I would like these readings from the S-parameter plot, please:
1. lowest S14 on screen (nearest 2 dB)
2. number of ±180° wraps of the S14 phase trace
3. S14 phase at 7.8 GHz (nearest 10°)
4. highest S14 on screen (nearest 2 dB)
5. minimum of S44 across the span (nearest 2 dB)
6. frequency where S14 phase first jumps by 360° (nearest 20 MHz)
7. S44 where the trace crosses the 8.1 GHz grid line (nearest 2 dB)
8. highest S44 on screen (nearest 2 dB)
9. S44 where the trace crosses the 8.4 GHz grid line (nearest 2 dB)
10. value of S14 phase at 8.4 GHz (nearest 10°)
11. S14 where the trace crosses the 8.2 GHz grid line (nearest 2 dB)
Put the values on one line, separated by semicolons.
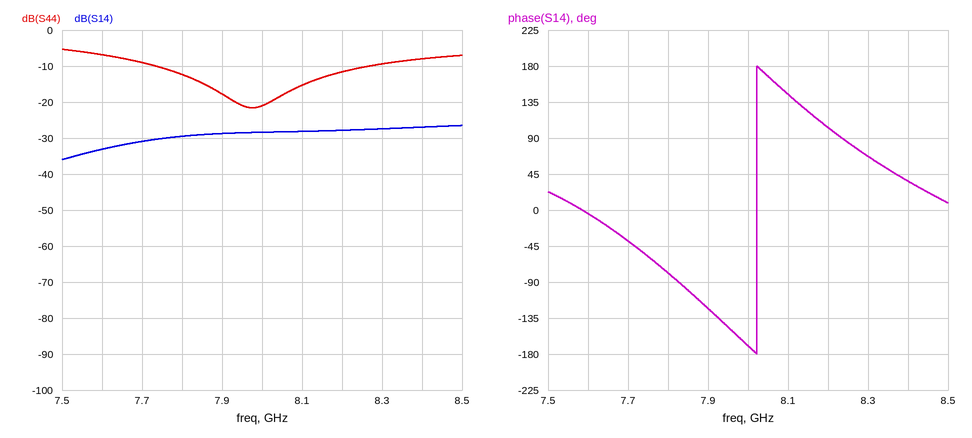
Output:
-36 dB; 1; -80°; -26 dB; -22 dB; 8.02 GHz; -16 dB; -6 dB; -8 dB; 40°; -28 dB
